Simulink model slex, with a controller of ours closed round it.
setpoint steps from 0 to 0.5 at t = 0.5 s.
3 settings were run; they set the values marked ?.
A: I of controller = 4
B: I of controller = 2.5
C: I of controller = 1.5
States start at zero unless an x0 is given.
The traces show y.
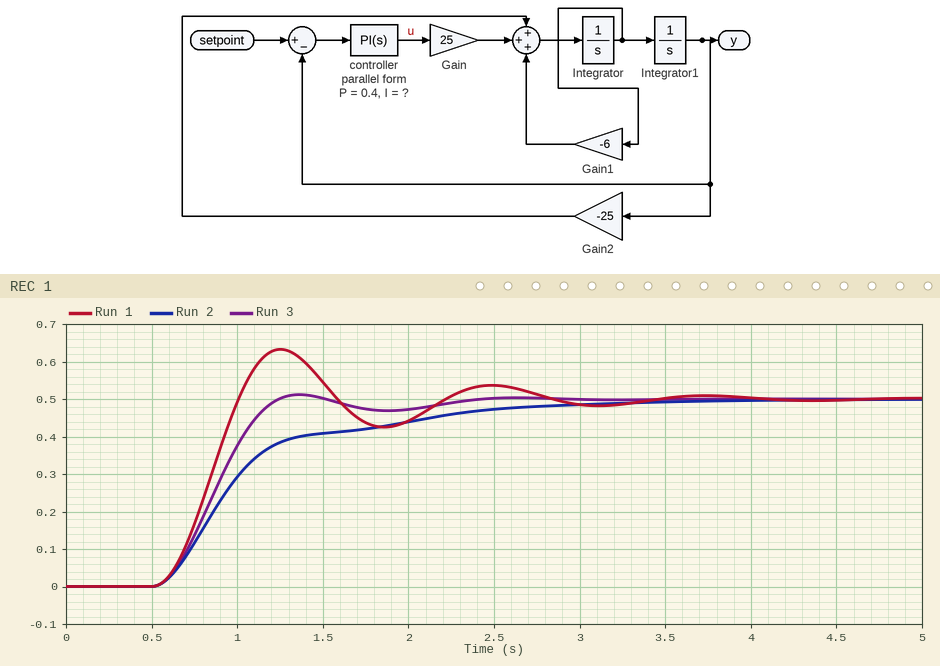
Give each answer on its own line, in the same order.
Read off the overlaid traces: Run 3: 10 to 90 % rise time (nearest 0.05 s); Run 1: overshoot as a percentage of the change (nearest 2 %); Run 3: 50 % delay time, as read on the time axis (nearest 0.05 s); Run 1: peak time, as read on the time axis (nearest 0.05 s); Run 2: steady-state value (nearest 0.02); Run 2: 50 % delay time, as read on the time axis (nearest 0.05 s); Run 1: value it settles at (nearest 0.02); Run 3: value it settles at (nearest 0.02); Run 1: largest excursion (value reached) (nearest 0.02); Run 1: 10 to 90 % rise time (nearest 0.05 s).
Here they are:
0.45 s
26 %
0.85 s
1.25 s
0.50
0.95 s
0.50
0.50
0.64
0.35 s
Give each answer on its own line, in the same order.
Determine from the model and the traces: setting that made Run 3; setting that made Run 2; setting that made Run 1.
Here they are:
B
C
A
